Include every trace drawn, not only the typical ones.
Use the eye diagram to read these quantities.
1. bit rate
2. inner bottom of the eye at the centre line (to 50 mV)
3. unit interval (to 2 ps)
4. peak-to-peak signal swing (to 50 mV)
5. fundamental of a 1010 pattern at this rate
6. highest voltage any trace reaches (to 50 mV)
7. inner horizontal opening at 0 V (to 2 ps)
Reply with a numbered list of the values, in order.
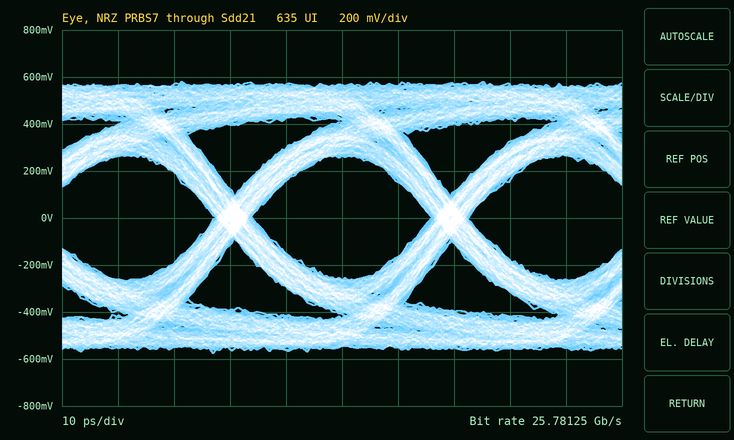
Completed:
1. 25.78125 Gb/s
2. -250 mV
3. 38 ps
4. 1.15 V
5. 12.89062 GHz
6. 600 mV
7. 32 ps
